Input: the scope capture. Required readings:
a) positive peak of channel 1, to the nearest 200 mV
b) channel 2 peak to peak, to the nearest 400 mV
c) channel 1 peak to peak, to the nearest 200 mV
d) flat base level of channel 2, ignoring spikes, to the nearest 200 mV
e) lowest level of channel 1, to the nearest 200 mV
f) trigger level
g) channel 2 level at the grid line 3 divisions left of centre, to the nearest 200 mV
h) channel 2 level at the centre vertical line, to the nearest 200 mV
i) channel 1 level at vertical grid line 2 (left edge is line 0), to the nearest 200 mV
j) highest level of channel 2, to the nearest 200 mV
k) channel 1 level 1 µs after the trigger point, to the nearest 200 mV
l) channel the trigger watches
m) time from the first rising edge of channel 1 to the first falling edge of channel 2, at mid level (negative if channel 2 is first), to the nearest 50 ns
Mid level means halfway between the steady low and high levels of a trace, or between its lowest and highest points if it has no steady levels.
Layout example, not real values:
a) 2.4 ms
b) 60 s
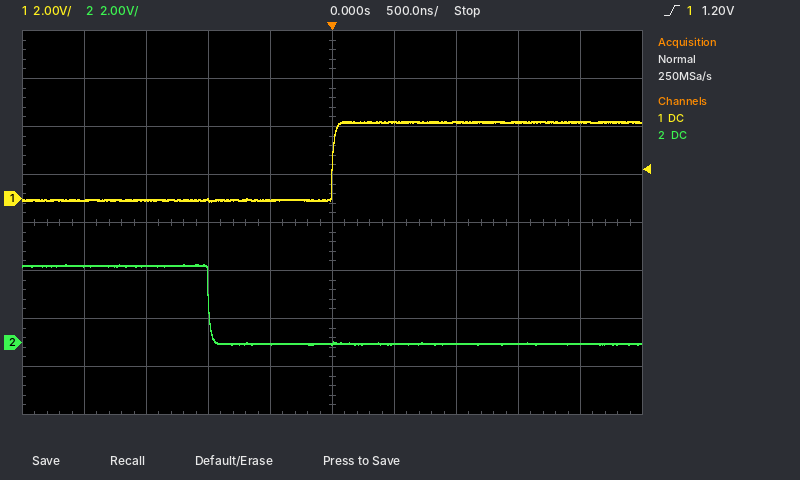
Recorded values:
a) 3.2 V
b) 3.2 V
c) 3.4 V
d) 0.0 V
e) -200 mV
f) 1.20 V
g) 3.2 V
h) 0.0 V
i) 0.0 V
j) 3.2 V
k) 3.2 V
l) channel 1
m) -1.00 µs
